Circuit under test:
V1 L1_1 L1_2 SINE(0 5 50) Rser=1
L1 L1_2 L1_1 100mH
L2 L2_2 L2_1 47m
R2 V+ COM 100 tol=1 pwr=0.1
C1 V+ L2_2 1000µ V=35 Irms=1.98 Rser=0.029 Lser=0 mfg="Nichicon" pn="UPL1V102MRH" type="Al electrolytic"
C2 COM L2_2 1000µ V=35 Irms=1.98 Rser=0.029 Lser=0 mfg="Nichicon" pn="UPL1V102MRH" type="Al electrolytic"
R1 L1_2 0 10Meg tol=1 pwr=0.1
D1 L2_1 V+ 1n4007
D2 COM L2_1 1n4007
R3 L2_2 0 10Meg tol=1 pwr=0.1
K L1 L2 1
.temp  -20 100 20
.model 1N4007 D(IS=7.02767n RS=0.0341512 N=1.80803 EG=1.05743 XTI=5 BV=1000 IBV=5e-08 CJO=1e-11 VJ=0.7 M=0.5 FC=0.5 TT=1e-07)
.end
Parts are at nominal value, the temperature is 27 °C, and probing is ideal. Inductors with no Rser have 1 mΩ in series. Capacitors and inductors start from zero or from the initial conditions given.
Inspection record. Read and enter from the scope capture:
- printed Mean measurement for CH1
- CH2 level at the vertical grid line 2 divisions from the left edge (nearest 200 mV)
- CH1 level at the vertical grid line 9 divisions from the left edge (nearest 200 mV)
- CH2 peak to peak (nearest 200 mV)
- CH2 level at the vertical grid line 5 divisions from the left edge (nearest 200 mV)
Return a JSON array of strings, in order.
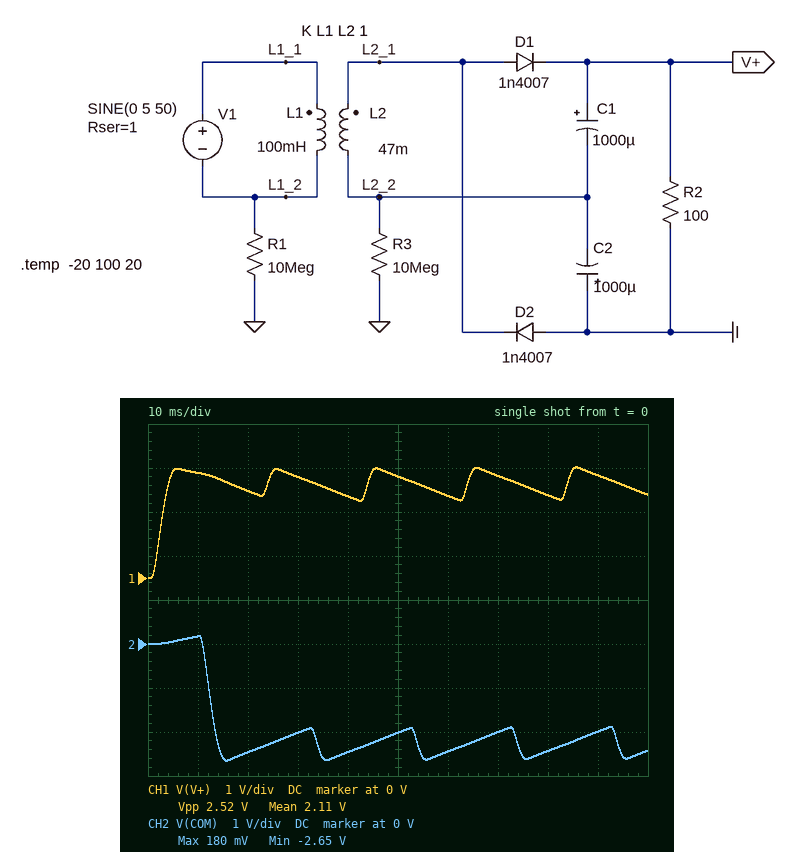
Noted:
["2.11 V", "-2.4 V", "2.4 V", "2.8 V", "-2.0 V"]
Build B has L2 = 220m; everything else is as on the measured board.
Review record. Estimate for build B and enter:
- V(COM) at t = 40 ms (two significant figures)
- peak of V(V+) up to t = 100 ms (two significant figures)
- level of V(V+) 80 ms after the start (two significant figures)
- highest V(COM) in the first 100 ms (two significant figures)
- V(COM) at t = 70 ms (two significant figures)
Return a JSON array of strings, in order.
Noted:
["-5.4 V", "5.5 V", "4.2 V", "330 mV", "-4.5 V"]
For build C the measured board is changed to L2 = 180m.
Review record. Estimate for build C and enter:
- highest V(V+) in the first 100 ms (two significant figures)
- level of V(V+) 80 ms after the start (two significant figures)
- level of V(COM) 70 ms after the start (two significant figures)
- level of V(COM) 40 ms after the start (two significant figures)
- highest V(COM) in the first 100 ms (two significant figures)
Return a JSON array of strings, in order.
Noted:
["5.1 V", "3.8 V", "-4.1 V", "-5.0 V", "320 mV"]
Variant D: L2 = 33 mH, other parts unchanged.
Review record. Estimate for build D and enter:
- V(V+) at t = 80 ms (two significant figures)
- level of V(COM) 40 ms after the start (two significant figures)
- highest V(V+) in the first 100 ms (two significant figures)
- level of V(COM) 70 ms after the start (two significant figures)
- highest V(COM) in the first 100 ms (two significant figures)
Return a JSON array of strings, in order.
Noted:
["1.5 V", "-2.0 V", "2.0 V", "-1.6 V", "140 mV"]
